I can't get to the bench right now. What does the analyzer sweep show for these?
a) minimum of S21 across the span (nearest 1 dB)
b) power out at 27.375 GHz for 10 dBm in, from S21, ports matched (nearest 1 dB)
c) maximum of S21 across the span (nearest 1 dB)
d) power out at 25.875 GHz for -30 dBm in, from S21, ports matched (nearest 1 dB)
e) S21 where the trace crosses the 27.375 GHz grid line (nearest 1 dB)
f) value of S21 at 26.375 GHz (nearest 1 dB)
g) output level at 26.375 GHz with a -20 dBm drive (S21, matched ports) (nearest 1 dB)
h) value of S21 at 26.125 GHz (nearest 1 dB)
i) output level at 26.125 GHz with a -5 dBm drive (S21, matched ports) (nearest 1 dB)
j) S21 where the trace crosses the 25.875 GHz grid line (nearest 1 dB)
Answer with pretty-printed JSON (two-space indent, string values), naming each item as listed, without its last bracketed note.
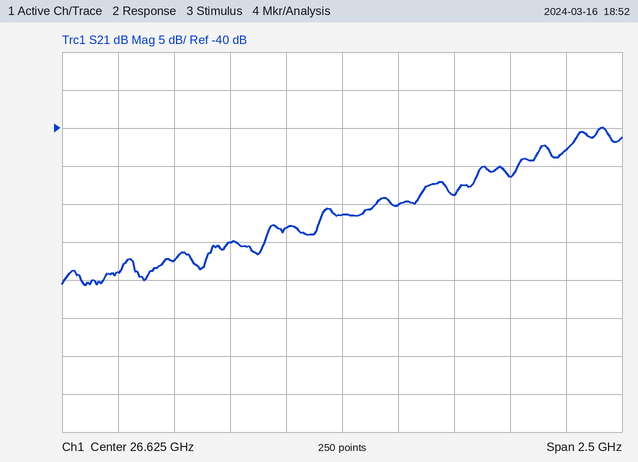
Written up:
{
  "minimum of S21 across the span": "-61 dB",
  "power out at 27.375 GHz for 10 dBm in, from S21, ports matched": "-36 dBm",
  "maximum of S21 across the span": "-40 dB",
  "power out at 25.875 GHz for -30 dBm in, from S21, ports matched": "-87 dBm",
  "S21 where the trace crosses the 27.375 GHz grid line": "-46 dB",
  "value of S21 at 26.375 GHz": "-53 dB",
  "output level at 26.375 GHz with a -20 dBm drive (S21, matched ports)": "-73 dBm",
  "value of S21 at 26.125 GHz": "-55 dB",
  "output level at 26.125 GHz with a -5 dBm drive (S21, matched ports)": "-60 dBm",
  "S21 where the trace crosses the 25.875 GHz grid line": "-57 dB"
}
